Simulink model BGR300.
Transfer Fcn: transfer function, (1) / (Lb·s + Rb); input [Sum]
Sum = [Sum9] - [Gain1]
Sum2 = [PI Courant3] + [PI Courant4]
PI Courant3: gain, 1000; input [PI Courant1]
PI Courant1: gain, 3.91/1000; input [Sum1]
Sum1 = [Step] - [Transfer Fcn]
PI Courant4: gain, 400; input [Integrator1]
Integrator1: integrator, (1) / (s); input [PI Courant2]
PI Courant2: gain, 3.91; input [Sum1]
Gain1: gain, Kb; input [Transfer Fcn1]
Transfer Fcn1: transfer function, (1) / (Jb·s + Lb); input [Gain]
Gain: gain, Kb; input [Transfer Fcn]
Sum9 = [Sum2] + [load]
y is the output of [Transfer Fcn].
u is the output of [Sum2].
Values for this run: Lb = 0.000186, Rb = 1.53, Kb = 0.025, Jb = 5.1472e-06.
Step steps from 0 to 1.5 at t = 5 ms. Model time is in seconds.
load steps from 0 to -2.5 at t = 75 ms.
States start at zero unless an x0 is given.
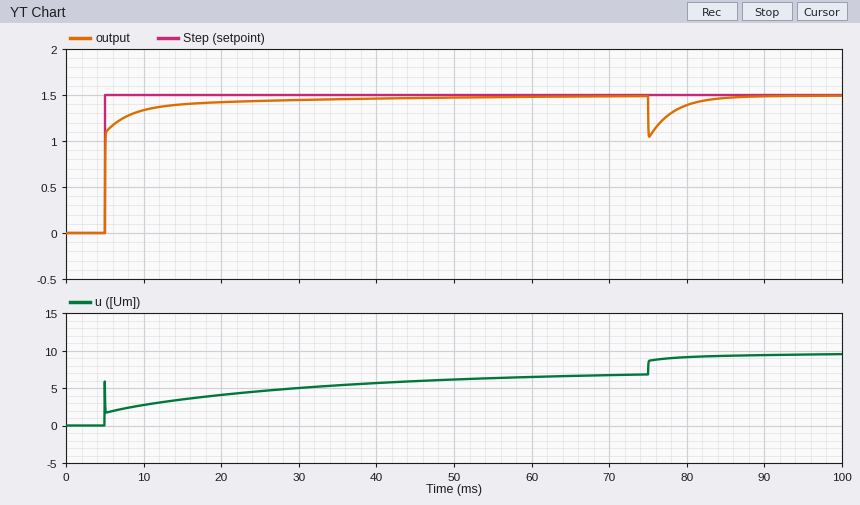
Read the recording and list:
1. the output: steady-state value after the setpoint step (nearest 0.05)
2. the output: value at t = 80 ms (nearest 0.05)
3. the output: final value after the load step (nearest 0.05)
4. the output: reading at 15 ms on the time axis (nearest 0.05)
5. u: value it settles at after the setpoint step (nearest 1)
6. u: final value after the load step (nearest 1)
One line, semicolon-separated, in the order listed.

1.50; 1.40; 1.50; 1.40; 7; 10
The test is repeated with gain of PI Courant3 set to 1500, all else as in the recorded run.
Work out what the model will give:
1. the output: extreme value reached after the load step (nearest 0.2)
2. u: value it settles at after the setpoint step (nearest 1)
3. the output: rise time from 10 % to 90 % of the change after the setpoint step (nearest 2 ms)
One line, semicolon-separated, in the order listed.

1.2; 7; 6 ms
